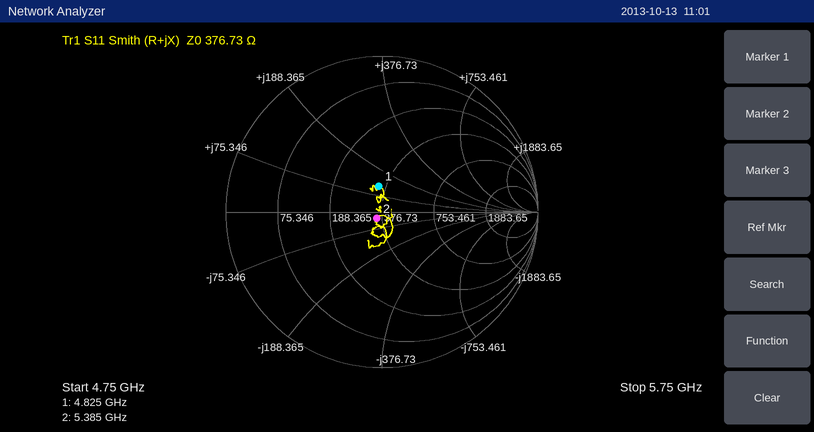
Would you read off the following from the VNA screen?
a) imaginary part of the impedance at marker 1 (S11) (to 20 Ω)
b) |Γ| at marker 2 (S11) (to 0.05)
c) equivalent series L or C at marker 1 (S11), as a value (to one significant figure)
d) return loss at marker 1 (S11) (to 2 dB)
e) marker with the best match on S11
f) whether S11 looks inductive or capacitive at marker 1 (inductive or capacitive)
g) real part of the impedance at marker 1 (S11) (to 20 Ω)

+120 Ω
0.05
4 nH
16 dB
marker 2
inductive
340 Ω
